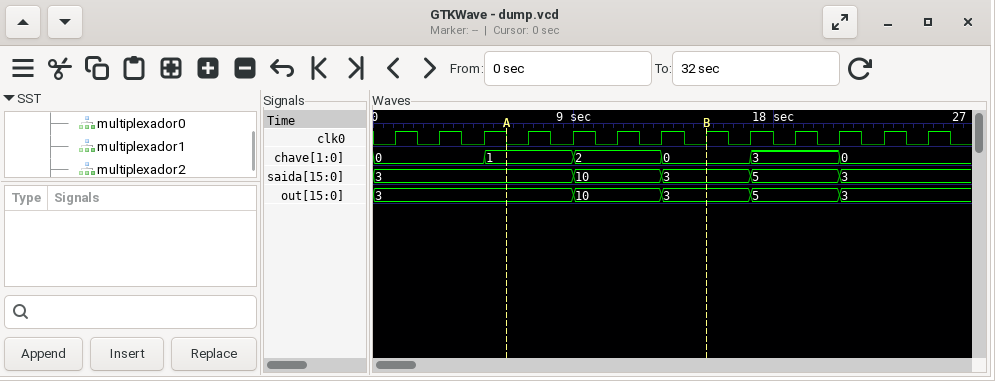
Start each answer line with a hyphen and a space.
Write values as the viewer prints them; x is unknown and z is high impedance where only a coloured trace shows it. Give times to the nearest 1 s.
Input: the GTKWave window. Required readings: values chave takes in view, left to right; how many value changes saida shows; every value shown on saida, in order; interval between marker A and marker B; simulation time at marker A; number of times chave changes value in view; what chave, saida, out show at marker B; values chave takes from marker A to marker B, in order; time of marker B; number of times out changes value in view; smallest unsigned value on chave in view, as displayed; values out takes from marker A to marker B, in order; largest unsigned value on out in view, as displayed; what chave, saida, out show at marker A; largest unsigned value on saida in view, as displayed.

- 0, 1, 2, 0, 3, 0
- 4
- 3, 10, 3, 5, 3
- 9 s
- 6 s
- 5
- chave=0, saida=3, out=3
- 1, 2, 0
- 15 s
- 4
- 0
- 3, 10, 3
- 10
- chave=1, saida=3, out=3
- 10
